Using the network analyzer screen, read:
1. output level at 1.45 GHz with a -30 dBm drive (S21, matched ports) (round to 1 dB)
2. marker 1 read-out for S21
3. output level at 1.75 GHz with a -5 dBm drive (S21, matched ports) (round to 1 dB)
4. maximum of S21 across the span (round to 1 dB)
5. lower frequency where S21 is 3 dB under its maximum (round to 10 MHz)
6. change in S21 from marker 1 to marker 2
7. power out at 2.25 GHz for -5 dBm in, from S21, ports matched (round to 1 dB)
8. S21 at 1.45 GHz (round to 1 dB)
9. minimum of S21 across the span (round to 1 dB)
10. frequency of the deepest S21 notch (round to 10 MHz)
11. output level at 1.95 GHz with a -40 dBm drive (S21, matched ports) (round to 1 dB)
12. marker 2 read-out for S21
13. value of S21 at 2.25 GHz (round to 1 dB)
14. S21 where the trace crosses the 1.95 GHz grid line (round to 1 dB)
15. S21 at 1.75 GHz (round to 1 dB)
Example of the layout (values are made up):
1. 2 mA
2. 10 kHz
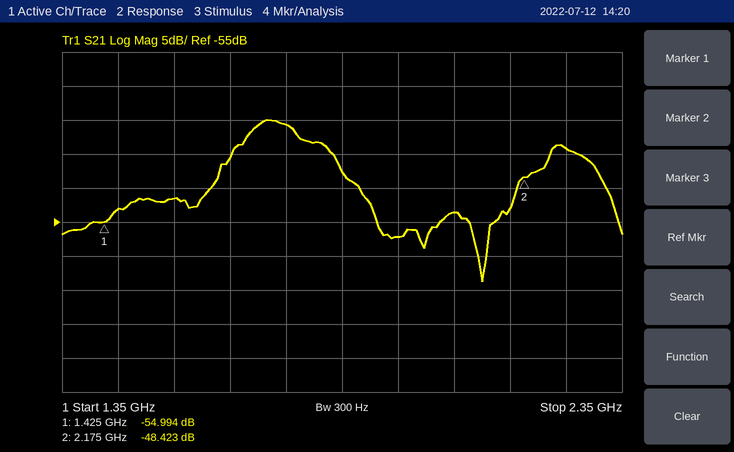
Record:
1. -83 dBm
2. -54.994 dB
3. -46 dBm
4. -40 dB
5. 1.68 GHz
6. 6.571 dB
7. -49 dBm
8. -53 dB
9. -64 dB
10. 2.10 GHz
11. -97 dBm
12. -48.423 dB
13. -44 dB
14. -57 dB
15. -41 dB
